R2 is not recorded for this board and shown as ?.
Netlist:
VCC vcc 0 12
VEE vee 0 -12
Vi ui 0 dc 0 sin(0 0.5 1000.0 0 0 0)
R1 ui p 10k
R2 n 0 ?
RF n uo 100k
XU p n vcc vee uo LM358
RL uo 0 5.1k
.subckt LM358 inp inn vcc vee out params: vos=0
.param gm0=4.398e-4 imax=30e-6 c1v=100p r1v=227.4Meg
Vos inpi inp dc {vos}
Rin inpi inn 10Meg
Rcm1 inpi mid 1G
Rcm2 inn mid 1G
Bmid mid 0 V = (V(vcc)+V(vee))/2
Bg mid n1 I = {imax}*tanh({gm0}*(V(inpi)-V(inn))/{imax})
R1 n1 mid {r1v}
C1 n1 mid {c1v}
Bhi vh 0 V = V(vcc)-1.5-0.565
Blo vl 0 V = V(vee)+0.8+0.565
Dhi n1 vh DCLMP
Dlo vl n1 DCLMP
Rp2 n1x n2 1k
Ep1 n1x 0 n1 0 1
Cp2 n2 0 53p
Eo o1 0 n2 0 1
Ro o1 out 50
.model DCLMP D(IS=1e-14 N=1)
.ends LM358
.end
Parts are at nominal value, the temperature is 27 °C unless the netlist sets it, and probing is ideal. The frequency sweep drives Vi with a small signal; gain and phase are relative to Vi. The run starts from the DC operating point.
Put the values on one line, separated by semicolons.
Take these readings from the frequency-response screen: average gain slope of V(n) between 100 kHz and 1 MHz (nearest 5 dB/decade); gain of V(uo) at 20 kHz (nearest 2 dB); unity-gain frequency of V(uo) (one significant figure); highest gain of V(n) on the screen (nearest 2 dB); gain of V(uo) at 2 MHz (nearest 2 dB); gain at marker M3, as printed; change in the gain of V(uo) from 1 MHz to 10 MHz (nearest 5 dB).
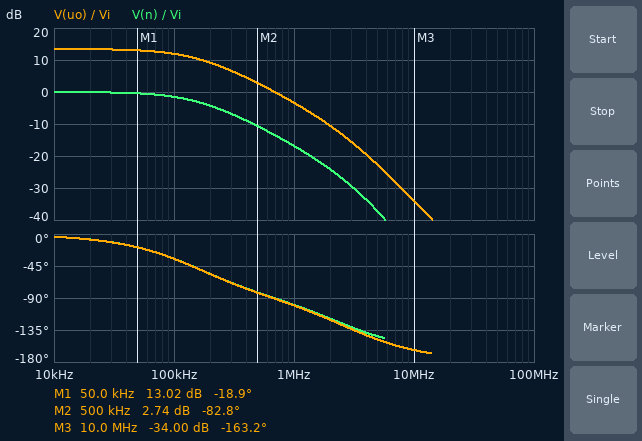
-15 dB/decade; 14 dB; 700 kHz; 0 dB; -10 dB; -34.00 dB; -30 dB
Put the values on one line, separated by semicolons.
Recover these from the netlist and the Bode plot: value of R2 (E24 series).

27 kΩ
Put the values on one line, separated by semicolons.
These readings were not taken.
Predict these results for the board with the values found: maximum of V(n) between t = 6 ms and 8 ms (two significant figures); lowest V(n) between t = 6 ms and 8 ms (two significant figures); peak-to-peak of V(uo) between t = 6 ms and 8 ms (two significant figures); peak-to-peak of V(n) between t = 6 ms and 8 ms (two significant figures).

500 mV; -500 mV; 4.7 V; 1.0 V
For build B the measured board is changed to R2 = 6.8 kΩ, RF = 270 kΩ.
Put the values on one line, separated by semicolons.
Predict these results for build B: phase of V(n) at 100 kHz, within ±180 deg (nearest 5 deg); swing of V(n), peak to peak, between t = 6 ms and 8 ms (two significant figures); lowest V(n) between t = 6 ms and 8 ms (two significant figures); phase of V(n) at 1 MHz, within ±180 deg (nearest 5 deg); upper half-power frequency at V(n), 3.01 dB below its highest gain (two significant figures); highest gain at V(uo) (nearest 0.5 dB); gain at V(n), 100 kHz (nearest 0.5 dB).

-80 deg; 530 mV; -270 mV; -105 deg; 17 kHz; 32.0 dB; -15.5 dB
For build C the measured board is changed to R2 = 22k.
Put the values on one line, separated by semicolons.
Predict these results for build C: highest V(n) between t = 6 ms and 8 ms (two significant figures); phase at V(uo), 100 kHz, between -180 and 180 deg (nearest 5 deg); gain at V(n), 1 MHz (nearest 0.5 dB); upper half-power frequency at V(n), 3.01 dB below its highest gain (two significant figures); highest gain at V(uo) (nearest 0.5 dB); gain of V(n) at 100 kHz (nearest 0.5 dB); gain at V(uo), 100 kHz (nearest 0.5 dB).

500 mV; -40 deg; -18.5 dB; 130 kHz; 15.0 dB; -2.0 dB; 13.0 dB
